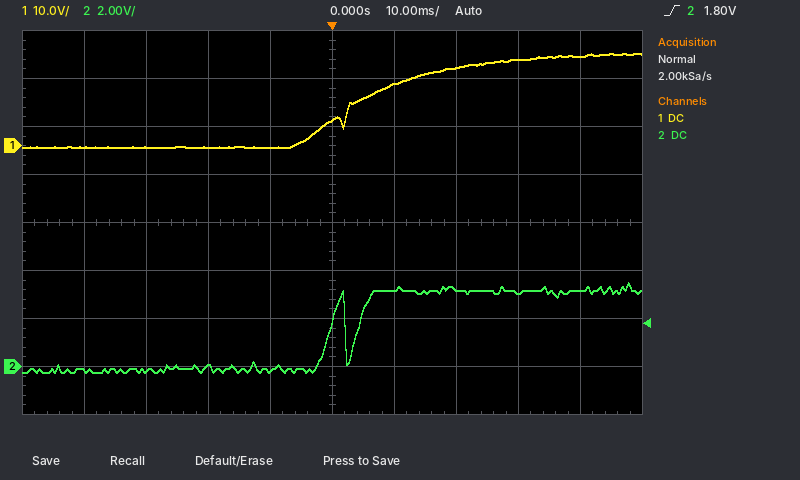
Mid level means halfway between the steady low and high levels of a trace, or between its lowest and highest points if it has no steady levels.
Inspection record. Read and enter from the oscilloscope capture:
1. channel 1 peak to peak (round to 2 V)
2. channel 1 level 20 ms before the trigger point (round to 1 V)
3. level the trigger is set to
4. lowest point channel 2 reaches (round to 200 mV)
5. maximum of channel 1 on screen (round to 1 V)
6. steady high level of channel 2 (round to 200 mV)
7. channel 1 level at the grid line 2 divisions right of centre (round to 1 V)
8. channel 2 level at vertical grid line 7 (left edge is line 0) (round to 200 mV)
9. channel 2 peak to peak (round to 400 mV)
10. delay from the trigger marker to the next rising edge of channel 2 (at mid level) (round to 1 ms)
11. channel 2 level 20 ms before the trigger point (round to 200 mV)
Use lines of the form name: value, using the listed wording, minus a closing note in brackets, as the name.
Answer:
channel 1 peak to peak: 20 V
channel 1 level 20 ms before the trigger point: 0 V
level the trigger is set to: 1.80 V
lowest point channel 2 reaches: -200 mV
maximum of channel 1 on screen: 19 V
steady high level of channel 2: 3.2 V
channel 1 level at the grid line 2 divisions right of centre: 16 V
channel 2 level at vertical grid line 7 (left edge is line 0): 3.2 V
channel 2 peak to peak: 3.6 V
delay from the trigger marker to the next rising edge of channel 2 (at mid level): 4 ms
channel 2 level 20 ms before the trigger point: 0.0 V
